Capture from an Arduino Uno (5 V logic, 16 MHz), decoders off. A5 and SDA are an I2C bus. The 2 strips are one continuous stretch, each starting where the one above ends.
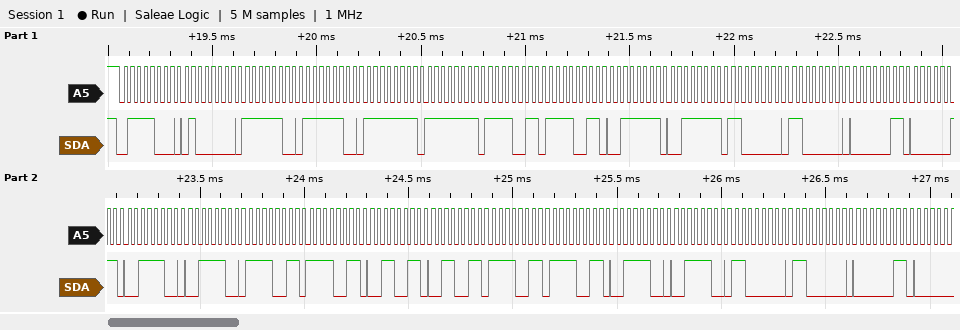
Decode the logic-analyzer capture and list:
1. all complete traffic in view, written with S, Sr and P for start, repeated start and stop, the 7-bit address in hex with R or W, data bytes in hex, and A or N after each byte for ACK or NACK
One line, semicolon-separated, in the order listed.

S 3CW A 40 A FC A FC A FF A FF A F3 A F3 A 3F A 3F A C0 A C0 A 03 A 03 A 3C A 3C A F3 A F3 A 33 A 33 A F3 A F3 A 3C A 3C A C0 A C0 A 03 A
